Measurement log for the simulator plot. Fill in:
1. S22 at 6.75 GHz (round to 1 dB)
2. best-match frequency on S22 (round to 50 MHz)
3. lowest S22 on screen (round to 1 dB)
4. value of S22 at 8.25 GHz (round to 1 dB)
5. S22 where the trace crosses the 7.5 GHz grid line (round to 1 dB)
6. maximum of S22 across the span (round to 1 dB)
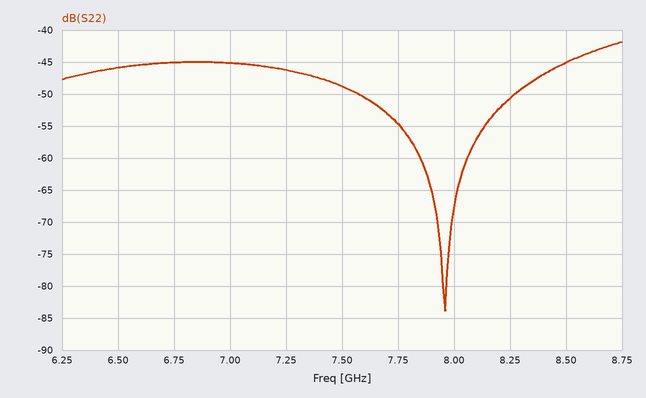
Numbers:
-45 dB
7.95 GHz
-84 dB
-51 dB
-49 dB
-42 dB
